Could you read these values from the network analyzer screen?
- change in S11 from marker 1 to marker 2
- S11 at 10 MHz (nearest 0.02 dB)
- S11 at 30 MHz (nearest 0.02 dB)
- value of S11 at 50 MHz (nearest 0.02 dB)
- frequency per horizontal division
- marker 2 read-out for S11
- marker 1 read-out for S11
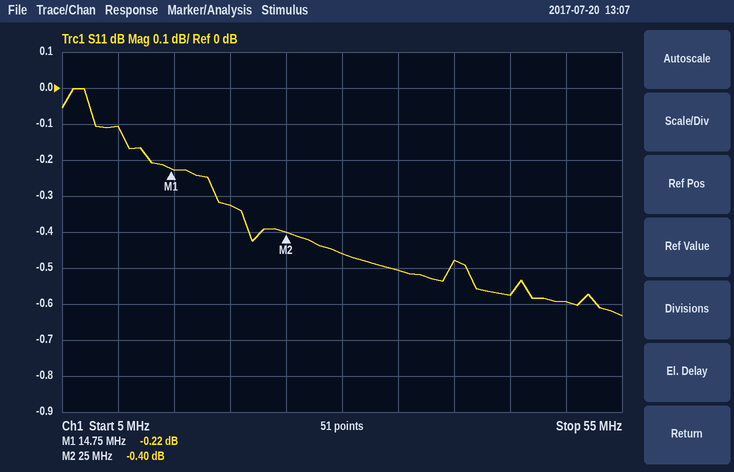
-0.18 dB
-0.10 dB
-0.46 dB
-0.60 dB
5 MHz
-0.40 dB
-0.22 dB
